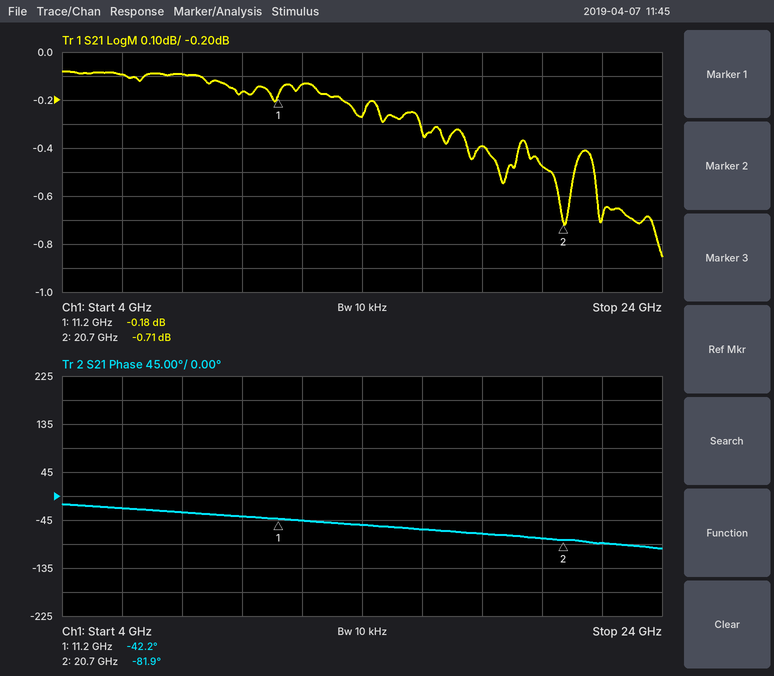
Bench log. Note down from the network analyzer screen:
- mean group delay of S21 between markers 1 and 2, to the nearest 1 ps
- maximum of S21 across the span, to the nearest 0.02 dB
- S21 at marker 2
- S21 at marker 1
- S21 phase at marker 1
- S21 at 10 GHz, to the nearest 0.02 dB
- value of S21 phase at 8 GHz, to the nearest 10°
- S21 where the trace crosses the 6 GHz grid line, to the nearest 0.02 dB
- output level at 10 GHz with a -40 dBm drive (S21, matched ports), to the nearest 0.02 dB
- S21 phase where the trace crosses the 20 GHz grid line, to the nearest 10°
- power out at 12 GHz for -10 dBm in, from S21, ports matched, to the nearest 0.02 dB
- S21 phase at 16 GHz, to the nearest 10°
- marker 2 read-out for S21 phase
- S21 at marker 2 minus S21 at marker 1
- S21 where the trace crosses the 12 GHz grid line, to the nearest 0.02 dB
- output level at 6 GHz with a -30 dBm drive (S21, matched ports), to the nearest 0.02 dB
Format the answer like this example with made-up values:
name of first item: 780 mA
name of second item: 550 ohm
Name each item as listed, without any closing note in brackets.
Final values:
mean group delay of S21 between markers 1 and 2, to the nearest 1 ps: 12 ps
maximum of S21 across the span, to the nearest 0.02 dB: -0.08 dB
S21 at marker 2: -0.71 dB
S21 at marker 1: -0.18 dB
S21 phase at marker 1: -42.2°
S21 at 10 GHz, to the nearest 0.02 dB: -0.16 dB
value of S21 phase at 8 GHz, to the nearest 10°: -30°
S21 where the trace crosses the 6 GHz grid line, to the nearest 0.02 dB: -0.10 dB
output level at 10 GHz with a -40 dBm drive (S21, matched ports), to the nearest 0.02 dB: -40.16 dBm
S21 phase where the trace crosses the 20 GHz grid line, to the nearest 10°: -80°
power out at 12 GHz for -10 dBm in, from S21, ports matched, to the nearest 0.02 dB: -10.14 dBm
S21 phase at 16 GHz, to the nearest 10°: -60°
marker 2 read-out for S21 phase: -81.9°
S21 at marker 2 minus S21 at marker 1: -0.53 dB
S21 where the trace crosses the 12 GHz grid line, to the nearest 0.02 dB: -0.14 dB
output level at 6 GHz with a -30 dBm drive (S21, matched ports), to the nearest 0.02 dB: -30.10 dBm
